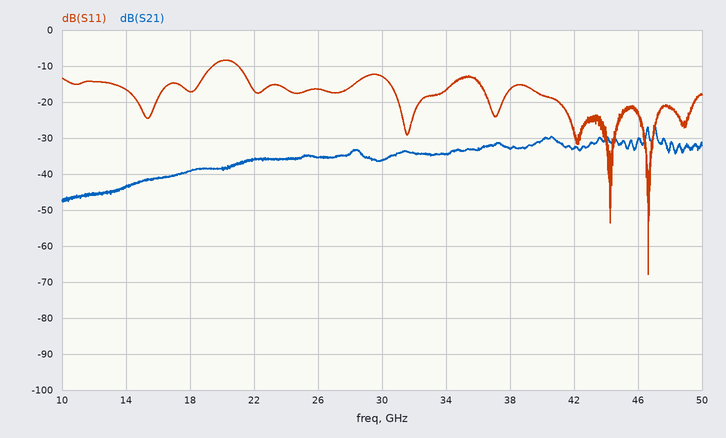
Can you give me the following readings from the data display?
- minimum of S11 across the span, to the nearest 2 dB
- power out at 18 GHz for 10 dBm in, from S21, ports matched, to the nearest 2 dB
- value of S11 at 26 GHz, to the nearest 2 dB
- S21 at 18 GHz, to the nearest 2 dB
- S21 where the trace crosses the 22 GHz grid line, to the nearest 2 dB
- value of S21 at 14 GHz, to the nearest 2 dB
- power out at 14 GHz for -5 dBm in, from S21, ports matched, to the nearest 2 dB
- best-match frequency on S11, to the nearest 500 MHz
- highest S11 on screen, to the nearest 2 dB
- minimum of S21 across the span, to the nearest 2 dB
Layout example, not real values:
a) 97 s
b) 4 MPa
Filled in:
a) -68 dB
b) -30 dBm
c) -16 dB
d) -40 dB
e) -36 dB
f) -44 dB
g) -48 dBm
h) 46.5 GHz
i) -8 dB
j) -48 dB
